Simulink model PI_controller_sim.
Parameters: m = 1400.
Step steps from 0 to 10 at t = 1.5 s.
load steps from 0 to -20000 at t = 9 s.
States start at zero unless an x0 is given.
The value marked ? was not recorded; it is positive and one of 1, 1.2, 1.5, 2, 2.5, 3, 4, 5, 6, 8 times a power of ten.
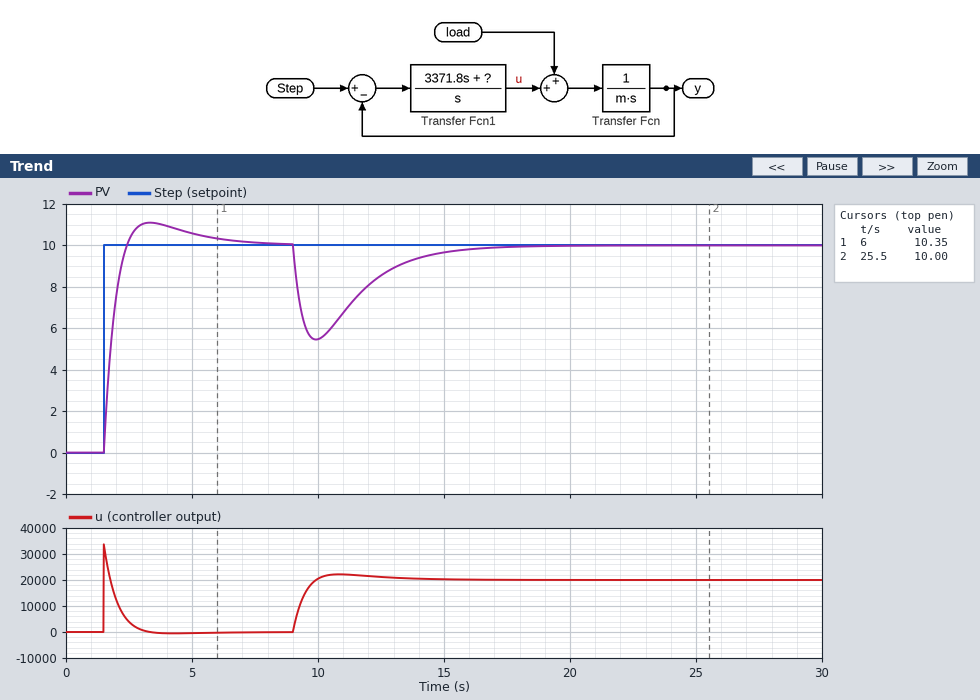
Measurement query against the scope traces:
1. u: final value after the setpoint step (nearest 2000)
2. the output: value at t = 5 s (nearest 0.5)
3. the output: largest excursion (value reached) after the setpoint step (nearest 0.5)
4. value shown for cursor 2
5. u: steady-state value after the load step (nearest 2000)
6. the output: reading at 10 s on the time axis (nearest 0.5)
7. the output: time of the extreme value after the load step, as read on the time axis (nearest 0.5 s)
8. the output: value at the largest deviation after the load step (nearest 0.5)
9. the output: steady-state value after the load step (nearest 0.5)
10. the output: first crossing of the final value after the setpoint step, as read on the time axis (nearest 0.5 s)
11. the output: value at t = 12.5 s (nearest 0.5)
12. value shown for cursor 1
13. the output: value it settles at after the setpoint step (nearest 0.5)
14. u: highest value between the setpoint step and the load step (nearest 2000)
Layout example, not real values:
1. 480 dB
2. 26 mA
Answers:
1. 0
2. 10.5
3. 11.0
4. 10.00
5. 20000
6. 5.5
7. 10.0 s
8. 5.5
9. 10.0
10. 2.5 s
11. 8.5
12. 10.35
13. 10.0
14. 34000
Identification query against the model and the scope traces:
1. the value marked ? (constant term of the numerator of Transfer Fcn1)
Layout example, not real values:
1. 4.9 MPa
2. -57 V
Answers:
1. 1500
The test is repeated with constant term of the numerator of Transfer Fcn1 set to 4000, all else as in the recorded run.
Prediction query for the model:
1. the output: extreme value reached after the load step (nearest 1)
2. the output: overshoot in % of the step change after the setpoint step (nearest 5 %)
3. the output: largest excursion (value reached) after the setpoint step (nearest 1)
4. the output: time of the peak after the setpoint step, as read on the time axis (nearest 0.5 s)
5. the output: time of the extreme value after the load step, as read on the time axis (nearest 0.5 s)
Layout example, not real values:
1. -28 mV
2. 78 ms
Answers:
1. 6
2. 20 %
3. 12
4. 3.0 s
5. 9.5 s
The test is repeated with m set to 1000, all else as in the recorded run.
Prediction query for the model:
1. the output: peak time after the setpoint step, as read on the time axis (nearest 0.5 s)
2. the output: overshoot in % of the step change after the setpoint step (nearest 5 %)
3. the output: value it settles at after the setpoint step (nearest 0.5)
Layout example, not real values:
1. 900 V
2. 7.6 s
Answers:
1. 3.0 s
2. 10 %
3. 10.0
